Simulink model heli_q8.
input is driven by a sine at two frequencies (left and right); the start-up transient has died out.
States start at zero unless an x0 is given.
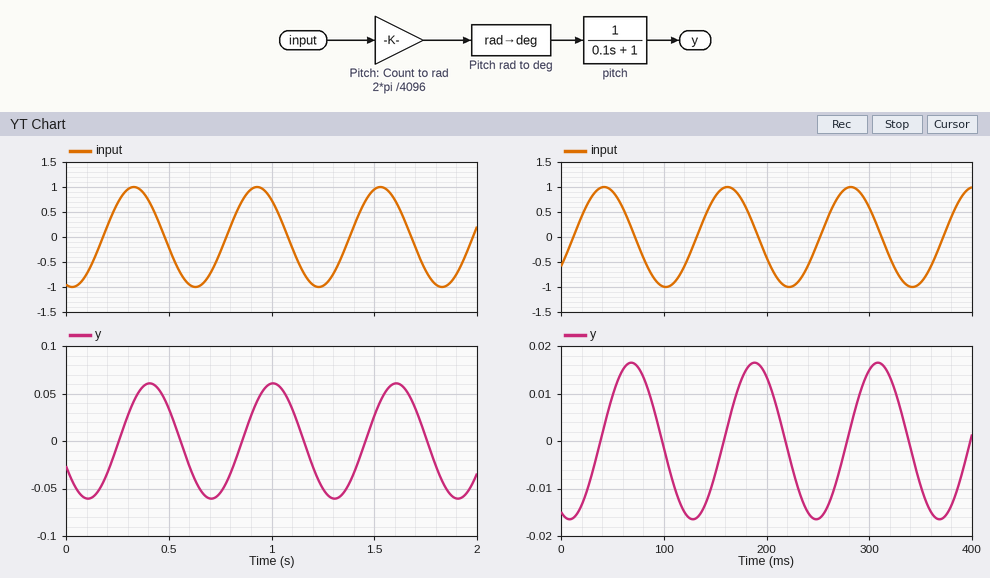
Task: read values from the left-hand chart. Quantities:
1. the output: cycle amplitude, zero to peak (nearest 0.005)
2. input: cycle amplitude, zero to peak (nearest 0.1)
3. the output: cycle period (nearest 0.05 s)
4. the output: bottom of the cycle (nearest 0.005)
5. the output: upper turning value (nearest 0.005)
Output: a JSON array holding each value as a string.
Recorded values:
["0.060", "1.0", "0.60 s", "-0.060", "0.060"]
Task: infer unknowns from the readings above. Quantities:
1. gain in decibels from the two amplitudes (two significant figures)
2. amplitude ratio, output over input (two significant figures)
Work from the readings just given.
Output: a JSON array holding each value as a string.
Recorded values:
["-24 dB", "0.060"]
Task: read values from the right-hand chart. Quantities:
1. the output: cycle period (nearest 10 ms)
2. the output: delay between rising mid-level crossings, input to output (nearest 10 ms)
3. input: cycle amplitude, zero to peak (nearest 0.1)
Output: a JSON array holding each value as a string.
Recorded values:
["120 ms", "30 ms", "1.0"]
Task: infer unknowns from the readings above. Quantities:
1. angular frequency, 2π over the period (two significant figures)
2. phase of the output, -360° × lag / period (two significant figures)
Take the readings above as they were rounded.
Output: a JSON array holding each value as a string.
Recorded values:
["0.052 rad/ms", "-90°"]
